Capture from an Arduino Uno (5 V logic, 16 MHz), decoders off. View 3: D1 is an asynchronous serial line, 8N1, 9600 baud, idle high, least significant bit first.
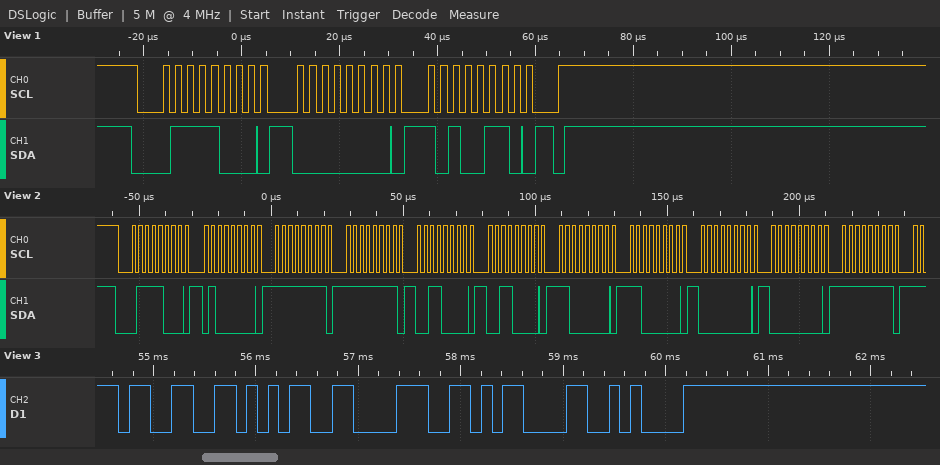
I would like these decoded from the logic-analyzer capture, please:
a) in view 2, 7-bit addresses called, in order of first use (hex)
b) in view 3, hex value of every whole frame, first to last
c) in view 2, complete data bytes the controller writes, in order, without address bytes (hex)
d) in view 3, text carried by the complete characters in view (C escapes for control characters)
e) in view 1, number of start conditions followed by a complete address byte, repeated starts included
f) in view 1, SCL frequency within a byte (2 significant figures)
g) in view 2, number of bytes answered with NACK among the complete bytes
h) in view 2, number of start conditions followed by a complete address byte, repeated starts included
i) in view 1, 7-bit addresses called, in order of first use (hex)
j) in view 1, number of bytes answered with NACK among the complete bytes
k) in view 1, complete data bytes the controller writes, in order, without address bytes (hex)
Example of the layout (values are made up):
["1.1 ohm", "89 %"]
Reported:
["0x3C", "33 35 38 0D 0A", "40 FF FF 30 30 C0 C0 00 00 FF", "\"358\\r\\n\"", "1", "400 kHz", "0", "1", "0x3C", "0", "00 A6"]
